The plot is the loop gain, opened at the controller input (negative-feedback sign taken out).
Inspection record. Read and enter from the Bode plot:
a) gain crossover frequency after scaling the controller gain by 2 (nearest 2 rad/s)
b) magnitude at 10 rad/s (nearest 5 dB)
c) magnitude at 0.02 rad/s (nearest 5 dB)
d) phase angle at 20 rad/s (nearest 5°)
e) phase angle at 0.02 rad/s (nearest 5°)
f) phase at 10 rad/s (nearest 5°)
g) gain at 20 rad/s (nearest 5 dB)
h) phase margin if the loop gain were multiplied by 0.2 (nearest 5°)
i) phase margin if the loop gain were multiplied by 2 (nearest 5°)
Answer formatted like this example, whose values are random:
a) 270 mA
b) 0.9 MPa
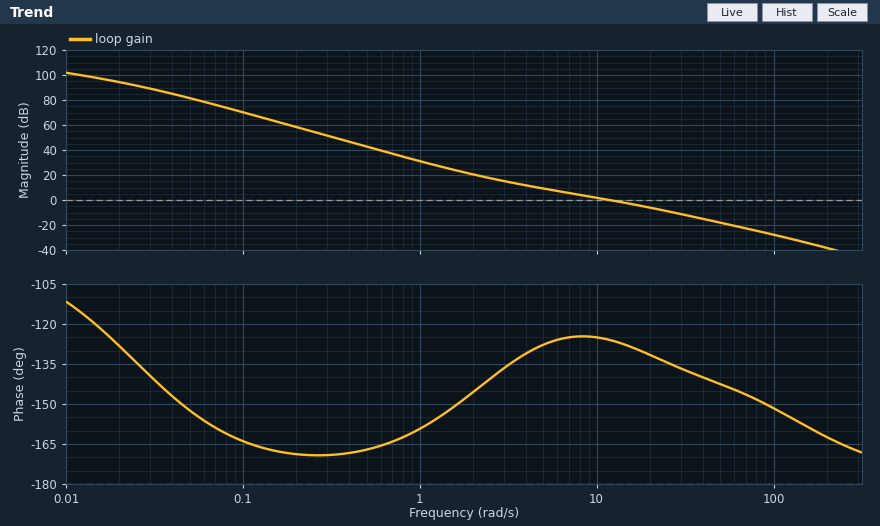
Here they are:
a) 20 rad/s
b) 0 dB
c) 95 dB
d) -130°
e) -130°
f) -125°
g) -5 dB
h) 45°
i) 50°
